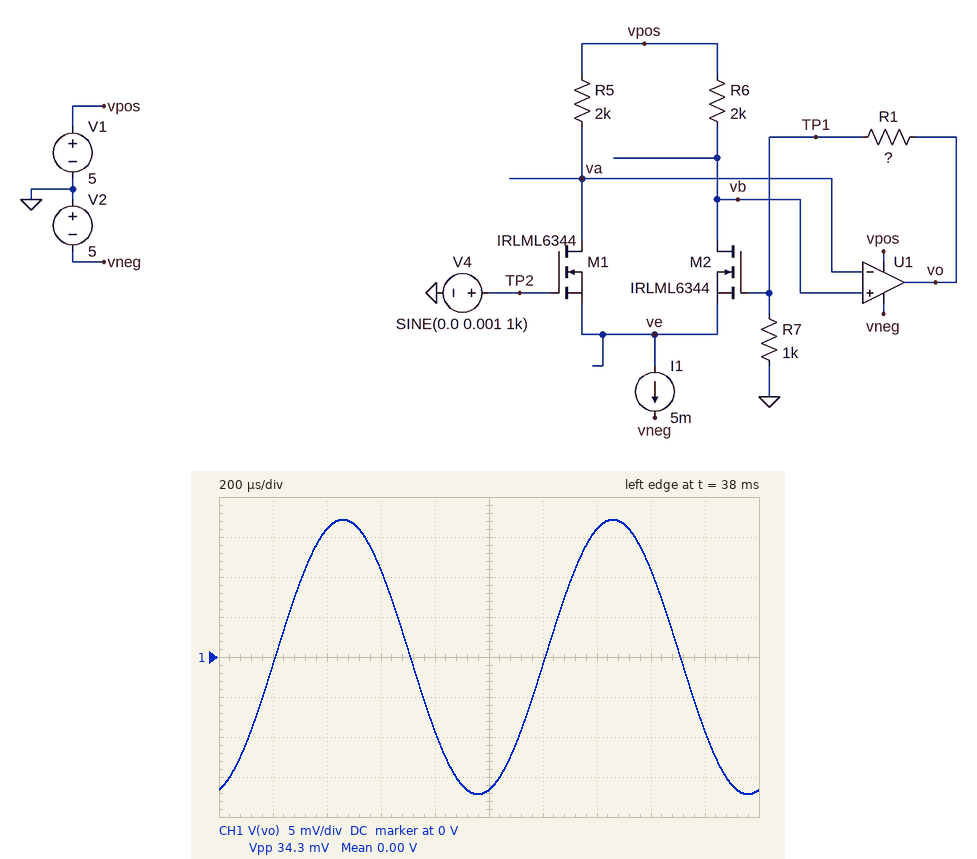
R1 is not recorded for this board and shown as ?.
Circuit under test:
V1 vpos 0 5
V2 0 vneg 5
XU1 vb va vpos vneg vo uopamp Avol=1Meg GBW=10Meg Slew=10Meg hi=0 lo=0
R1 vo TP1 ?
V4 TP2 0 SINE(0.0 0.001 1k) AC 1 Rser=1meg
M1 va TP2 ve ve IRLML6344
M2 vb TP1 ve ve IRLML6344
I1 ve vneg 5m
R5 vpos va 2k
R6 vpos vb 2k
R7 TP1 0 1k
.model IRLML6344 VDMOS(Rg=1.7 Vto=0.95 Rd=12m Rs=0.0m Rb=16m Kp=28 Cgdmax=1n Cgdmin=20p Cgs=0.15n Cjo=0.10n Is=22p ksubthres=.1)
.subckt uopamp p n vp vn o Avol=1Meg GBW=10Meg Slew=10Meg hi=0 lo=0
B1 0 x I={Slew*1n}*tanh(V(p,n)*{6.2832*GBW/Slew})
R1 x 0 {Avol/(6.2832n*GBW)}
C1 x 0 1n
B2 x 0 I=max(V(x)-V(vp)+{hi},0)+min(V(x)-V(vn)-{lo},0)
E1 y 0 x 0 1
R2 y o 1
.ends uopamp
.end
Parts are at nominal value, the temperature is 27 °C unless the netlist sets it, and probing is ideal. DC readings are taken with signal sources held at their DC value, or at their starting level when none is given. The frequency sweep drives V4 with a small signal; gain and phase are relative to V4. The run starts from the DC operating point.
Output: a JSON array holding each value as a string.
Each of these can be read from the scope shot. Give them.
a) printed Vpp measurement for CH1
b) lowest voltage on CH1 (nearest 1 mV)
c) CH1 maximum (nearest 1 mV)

["34.3 mV", "-17 mV", "17 mV"]
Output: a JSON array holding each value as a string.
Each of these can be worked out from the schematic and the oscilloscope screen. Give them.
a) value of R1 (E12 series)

["68 kΩ"]
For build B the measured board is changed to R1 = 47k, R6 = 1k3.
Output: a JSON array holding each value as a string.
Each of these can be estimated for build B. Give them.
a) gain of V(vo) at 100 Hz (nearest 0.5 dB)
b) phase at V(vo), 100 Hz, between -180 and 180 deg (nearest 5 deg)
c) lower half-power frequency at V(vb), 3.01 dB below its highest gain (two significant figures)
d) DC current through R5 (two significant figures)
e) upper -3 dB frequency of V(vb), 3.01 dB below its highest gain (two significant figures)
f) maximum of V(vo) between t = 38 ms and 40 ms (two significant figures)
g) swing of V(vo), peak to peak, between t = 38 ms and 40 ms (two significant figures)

["33.5 dB", "-10 deg", "64 kHz", "2.0 mA", "290 kHz", "1.1 V", "44 mV"]
